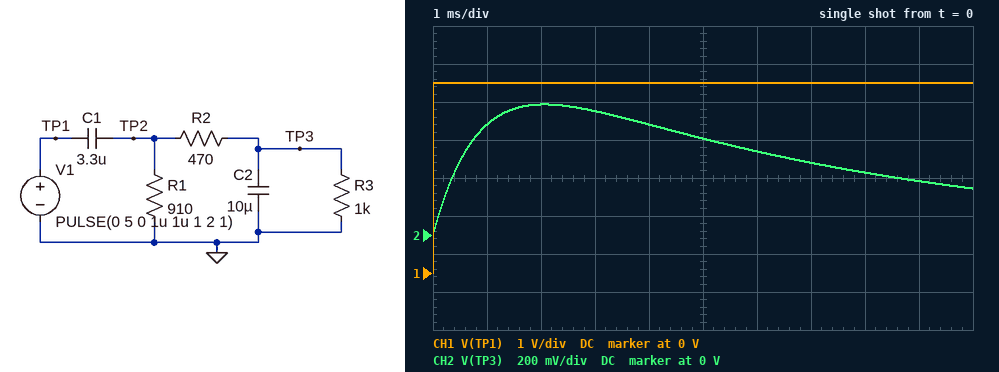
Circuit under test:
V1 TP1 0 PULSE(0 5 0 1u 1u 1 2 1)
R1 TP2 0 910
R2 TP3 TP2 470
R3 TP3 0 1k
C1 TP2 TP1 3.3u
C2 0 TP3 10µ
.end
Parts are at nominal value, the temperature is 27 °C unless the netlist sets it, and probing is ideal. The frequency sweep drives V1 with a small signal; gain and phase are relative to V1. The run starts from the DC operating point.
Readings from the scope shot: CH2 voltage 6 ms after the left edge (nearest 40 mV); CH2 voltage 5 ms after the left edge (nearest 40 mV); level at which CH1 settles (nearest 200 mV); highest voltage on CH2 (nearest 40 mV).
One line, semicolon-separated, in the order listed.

440 mV; 520 mV; 5.0 V; 680 mV
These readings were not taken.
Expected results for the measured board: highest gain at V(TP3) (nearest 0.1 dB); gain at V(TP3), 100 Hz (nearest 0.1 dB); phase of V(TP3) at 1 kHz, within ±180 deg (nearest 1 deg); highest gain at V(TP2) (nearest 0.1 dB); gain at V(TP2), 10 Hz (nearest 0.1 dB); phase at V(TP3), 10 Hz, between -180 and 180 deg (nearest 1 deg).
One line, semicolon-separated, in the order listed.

-15.7 dB; -16.0 dB; -78 deg; 0 dB; -19.2 dB; 64 deg
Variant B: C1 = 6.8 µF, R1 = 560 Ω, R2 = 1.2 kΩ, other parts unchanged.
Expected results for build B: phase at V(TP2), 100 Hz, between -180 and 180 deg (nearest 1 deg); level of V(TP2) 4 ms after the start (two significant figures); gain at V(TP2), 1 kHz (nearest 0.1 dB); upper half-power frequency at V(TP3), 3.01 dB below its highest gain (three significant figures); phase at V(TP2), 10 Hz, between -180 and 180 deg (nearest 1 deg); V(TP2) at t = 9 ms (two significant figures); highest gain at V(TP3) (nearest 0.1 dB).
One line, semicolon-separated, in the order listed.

31 deg; 1.2 V; 0 dB; 105 Hz; 77 deg; 300 mV; -16.7 dB
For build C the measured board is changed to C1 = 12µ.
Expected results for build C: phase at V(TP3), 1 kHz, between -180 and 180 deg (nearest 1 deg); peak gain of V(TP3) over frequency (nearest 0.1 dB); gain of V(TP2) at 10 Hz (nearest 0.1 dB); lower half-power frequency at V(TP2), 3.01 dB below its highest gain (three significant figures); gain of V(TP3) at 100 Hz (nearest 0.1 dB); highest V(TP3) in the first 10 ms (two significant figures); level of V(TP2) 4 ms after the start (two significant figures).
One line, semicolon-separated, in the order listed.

-85 deg; -8.7 dB; -8.9 dB; 44.3 Hz; -11.5 dB; 1.5 V; 2.2 V
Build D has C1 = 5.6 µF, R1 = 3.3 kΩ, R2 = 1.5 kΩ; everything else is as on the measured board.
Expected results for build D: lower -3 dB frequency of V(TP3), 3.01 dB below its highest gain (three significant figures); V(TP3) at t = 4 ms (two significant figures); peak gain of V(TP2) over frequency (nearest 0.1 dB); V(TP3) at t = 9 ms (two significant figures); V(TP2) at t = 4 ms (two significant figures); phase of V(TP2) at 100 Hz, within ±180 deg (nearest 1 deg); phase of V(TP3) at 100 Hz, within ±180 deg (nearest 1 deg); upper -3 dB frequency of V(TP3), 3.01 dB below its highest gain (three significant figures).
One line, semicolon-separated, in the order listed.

8.47 Hz; 690 mV; 0 dB; 720 mV; 2.7 V; 15 deg; -60 deg; 62.6 Hz
